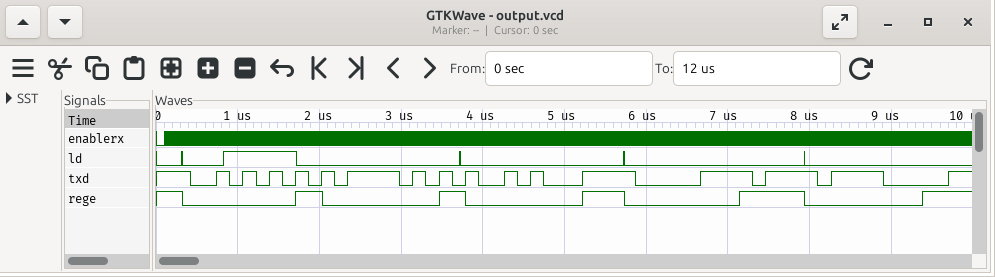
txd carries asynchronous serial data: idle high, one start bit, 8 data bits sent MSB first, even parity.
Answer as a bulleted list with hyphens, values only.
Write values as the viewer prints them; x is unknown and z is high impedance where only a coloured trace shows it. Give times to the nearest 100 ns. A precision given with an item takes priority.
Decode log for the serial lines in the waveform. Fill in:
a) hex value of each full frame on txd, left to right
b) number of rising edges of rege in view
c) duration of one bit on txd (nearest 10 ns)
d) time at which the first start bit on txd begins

- 55, F5, 51, 0F, F0
- 5
- 160 ns
- 400 ns
